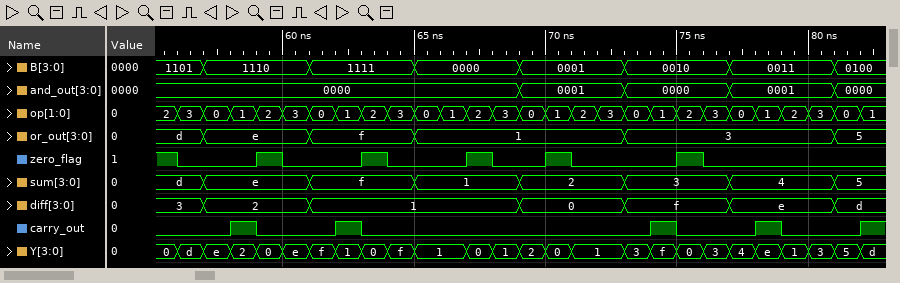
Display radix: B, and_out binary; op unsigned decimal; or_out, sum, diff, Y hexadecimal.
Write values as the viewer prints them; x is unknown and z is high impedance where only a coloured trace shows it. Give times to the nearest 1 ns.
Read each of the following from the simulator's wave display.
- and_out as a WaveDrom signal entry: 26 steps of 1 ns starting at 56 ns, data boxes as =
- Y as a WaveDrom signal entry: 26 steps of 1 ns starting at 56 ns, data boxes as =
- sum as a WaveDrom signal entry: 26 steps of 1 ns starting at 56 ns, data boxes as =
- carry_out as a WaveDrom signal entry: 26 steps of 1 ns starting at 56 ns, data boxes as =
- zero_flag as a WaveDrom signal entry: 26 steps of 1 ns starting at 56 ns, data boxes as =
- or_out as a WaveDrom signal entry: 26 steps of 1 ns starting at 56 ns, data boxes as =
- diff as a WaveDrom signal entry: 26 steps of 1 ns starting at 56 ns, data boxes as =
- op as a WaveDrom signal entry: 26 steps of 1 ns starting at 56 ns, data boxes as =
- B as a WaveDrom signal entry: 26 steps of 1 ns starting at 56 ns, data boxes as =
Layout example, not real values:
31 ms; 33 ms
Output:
{name: 'and_out', wave: '=............=...=...=...=', data: '0000 0001 0000 0001 0000'}; {name: 'Y', wave: '==========.=====.=========', data: 'd e 2 0 e f 1 0 f 1 0 1 2 0 1 3 f 0 3 4 e 1 3 5'}; {name: 'sum', wave: '==...=...=...=...=...=...=', data: 'd e f 1 2 3 4 5'}; {name: 'carry_out', wave: '0.10..10..........10..10..'}; {name: 'zero_flag', wave: '0..10..10..10.10...10.....'}; {name: 'or_out', wave: '==...=...=.......=.......=', data: 'd e f 1 3 5'}; {name: 'diff', wave: '==...=.......=...=...=...=', data: '3 2 1 0 f e d'}; {name: 'op', wave: '==========================', data: '3 0 1 2 3 0 1 2 3 0 1 2 3 0 1 2 3 0 1 2 3 0 1 2 3 0'}; {name: 'B', wave: '==...=...=...=...=...=...=', data: '1101 1110 1111 0000 0001 0010 0011 0100'}
